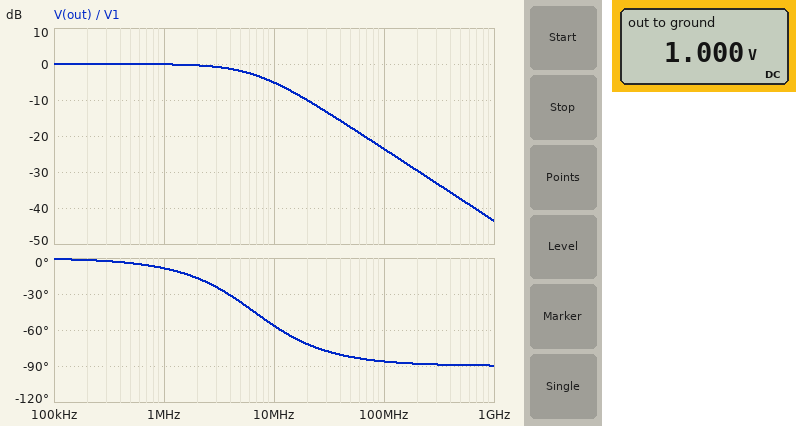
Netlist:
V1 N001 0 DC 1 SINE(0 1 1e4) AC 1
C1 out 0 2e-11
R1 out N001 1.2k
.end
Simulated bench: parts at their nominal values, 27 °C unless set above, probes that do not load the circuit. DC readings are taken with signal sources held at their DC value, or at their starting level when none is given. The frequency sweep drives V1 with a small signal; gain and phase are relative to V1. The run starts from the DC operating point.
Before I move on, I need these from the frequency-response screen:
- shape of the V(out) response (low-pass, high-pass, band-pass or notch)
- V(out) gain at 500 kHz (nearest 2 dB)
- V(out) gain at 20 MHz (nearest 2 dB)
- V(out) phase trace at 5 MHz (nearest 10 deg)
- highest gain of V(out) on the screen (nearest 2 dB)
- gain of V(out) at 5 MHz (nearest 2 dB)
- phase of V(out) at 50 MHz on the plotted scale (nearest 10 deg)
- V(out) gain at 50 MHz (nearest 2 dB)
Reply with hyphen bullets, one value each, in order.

- low-pass
- 0 dB
- -10 dB
- -40 deg
- 0 dB
- -2 dB
- -80 deg
- -18 dB
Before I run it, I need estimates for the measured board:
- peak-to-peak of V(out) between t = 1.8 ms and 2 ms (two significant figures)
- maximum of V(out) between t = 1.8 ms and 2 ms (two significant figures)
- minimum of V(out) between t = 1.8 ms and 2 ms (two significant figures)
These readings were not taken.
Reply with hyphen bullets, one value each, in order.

- 2.0 V
- 1.0 V
- -1.0 V
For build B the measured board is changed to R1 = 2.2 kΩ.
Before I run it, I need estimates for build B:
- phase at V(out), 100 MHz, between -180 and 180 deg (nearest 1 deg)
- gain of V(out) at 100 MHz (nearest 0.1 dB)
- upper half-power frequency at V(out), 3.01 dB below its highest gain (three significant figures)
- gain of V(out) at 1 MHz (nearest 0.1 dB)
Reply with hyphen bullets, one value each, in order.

- -88 deg
- -28.8 dB
- 3.62 MHz
- -0.3 dB
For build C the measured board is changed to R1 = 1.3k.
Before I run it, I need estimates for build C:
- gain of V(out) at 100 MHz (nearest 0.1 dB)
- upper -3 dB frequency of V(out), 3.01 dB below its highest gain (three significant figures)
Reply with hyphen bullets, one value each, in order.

- -24.3 dB
- 6.12 MHz
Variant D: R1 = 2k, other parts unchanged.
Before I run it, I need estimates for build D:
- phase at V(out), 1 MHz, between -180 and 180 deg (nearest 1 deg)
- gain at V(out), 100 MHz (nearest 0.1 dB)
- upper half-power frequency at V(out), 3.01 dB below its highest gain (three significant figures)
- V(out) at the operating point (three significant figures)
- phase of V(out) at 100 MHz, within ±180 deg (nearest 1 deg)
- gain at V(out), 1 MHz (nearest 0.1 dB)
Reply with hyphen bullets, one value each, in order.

- -14 deg
- -28.0 dB
- 3.98 MHz
- 1.00 V
- -88 deg
- -0.3 dB
